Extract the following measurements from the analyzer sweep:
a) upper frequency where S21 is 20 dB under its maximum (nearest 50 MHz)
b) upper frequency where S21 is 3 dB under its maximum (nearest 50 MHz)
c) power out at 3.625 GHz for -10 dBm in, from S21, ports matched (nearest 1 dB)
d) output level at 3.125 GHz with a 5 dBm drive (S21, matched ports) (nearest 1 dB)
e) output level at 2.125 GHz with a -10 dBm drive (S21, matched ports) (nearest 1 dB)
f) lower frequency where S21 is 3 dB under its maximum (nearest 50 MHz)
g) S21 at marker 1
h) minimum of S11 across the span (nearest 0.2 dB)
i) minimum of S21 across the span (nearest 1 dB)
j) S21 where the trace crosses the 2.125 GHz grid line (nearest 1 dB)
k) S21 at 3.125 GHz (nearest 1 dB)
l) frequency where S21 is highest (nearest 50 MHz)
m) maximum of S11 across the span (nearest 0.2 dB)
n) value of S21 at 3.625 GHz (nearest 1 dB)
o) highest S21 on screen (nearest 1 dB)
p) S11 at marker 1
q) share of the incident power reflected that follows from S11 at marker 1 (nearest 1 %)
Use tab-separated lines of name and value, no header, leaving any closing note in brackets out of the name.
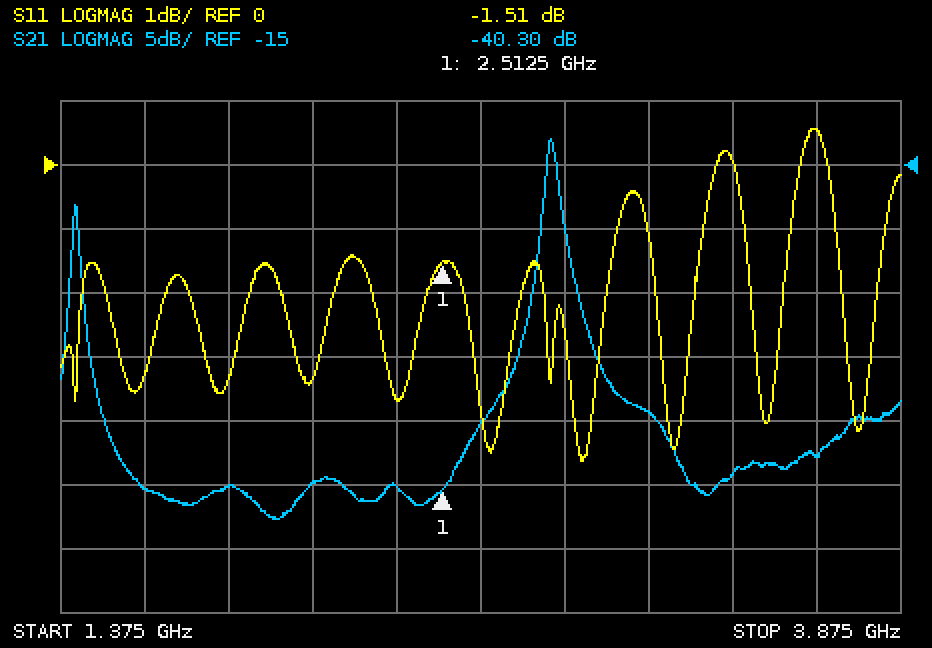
upper frequency where S21 is 20 dB under its maximum	3.05 GHz
upper frequency where S21 is 3 dB under its maximum	2.85 GHz
power out at 3.625 GHz for -10 dBm in, from S21, ports matched	-48 dBm
output level at 3.125 GHz with a 5 dBm drive (S21, matched ports)	-29 dBm
output level at 2.125 GHz with a -10 dBm drive (S21, matched ports)	-50 dBm
lower frequency where S21 is 3 dB under its maximum	2.80 GHz
S21 at marker 1	-40.30 dB
minimum of S11 across the span	-4.6 dB
minimum of S21 across the span	-43 dB
S21 where the trace crosses the 2.125 GHz grid line	-40 dB
S21 at 3.125 GHz	-34 dB
frequency where S21 is highest	2.85 GHz
maximum of S11 across the span	0.6 dB
value of S21 at 3.625 GHz	-38 dB
highest S21 on screen	-13 dB
S11 at marker 1	-1.51 dB
share of the incident power reflected that follows from S11 at marker 1	71 %
